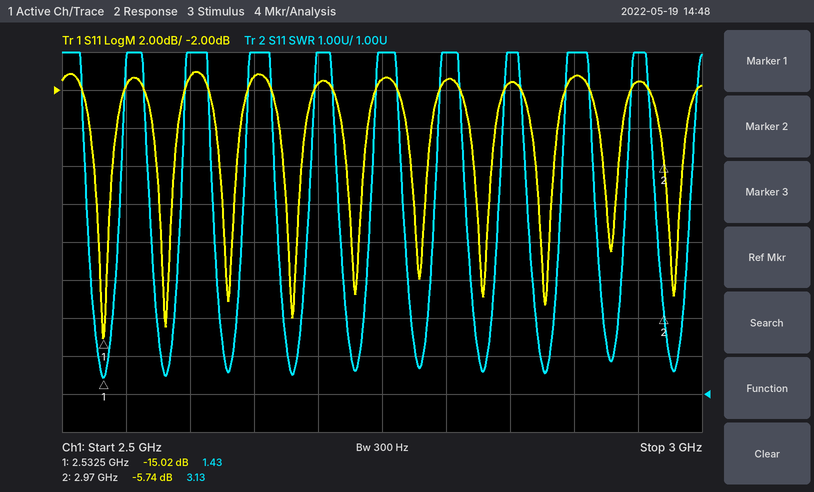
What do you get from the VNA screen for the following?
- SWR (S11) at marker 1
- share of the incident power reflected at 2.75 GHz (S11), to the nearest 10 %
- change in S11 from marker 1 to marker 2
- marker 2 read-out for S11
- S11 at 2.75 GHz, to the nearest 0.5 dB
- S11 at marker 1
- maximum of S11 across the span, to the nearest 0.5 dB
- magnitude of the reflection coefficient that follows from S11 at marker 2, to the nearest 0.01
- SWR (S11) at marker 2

1.43
70 %
9.28 dB
-5.74 dB
-1.5 dB
-15.02 dB
-1.0 dB
0.52
3.13
